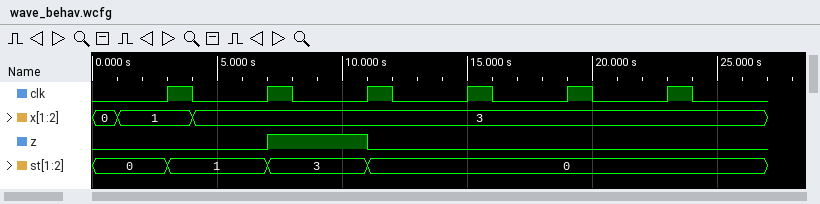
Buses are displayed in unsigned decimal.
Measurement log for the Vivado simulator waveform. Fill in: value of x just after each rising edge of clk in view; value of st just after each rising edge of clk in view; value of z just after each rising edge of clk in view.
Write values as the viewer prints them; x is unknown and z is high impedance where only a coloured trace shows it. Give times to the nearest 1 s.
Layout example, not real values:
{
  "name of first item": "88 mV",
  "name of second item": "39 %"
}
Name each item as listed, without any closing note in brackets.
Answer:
{
  "value of x just after each rising edge of clk in view": "1, 3, 3, 3, 3, 3",
  "value of st just after each rising edge of clk in view": "1, 3, 0, 0, 0, 0",
  "value of z just after each rising edge of clk in view": "0 1 0 0 0 0"
}
